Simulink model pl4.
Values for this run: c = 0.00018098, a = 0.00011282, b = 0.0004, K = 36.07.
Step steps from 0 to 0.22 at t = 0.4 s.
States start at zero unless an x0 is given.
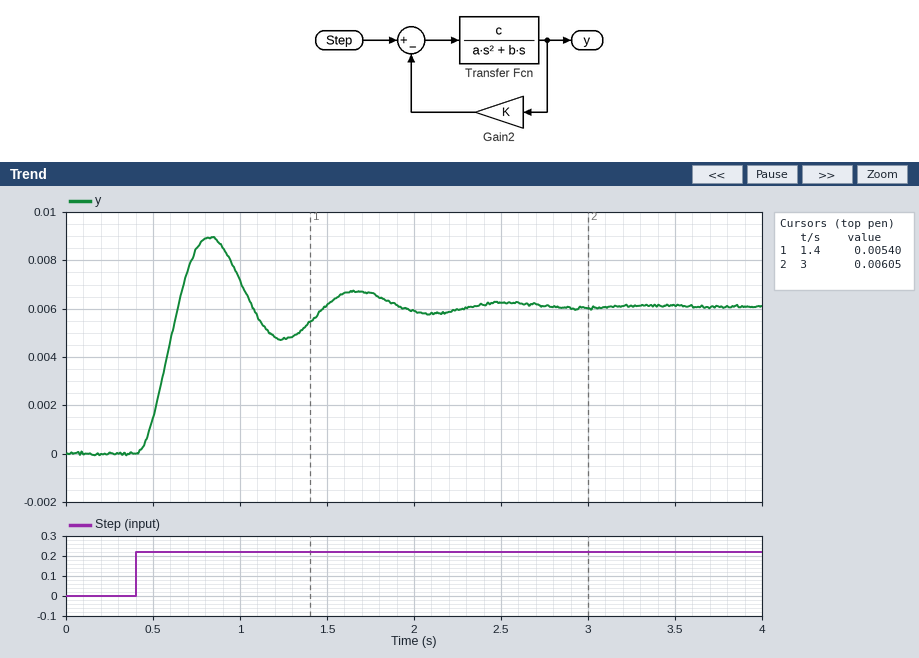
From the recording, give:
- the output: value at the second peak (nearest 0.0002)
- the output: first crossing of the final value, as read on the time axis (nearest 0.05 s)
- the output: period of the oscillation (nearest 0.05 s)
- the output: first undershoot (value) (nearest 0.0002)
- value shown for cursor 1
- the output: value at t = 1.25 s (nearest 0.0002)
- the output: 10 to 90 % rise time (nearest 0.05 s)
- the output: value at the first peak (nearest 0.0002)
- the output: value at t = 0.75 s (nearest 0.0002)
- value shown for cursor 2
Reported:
0.0068
0.65 s
0.85 s
0.0048
0.00540
0.0048
0.15 s
0.0090
0.0084
0.00605
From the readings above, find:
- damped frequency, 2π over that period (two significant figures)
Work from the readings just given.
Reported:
7.4 rad/s
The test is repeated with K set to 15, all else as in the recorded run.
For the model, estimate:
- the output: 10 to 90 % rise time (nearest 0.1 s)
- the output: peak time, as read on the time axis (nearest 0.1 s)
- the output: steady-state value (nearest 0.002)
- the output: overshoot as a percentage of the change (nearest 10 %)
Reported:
0.3 s
1.1 s
0.014
30 %
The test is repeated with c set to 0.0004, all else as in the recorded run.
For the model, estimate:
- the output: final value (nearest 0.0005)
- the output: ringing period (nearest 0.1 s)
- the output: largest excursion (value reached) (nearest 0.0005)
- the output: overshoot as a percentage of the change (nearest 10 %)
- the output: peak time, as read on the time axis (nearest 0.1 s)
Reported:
0.0060
0.6 s
0.0100
60 %
0.7 s
